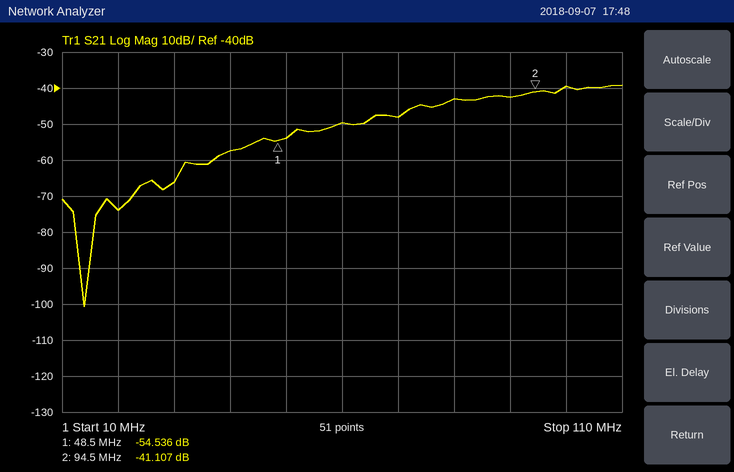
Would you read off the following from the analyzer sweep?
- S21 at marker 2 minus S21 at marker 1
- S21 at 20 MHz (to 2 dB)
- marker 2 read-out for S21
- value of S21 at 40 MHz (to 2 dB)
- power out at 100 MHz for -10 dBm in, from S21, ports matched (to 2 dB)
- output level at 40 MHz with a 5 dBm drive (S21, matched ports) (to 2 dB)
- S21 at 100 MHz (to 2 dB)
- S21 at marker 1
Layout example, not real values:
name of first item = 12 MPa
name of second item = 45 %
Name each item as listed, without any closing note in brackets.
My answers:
S21 at marker 2 minus S21 at marker 1 = 13.429 dB
S21 at 20 MHz = -74 dB
marker 2 read-out for S21 = -41.107 dB
value of S21 at 40 MHz = -58 dB
power out at 100 MHz for -10 dBm in, from S21, ports matched = -50 dBm
output level at 40 MHz with a 5 dBm drive (S21, matched ports) = -52 dBm
S21 at 100 MHz = -40 dB
S21 at marker 1 = -54.536 dB
